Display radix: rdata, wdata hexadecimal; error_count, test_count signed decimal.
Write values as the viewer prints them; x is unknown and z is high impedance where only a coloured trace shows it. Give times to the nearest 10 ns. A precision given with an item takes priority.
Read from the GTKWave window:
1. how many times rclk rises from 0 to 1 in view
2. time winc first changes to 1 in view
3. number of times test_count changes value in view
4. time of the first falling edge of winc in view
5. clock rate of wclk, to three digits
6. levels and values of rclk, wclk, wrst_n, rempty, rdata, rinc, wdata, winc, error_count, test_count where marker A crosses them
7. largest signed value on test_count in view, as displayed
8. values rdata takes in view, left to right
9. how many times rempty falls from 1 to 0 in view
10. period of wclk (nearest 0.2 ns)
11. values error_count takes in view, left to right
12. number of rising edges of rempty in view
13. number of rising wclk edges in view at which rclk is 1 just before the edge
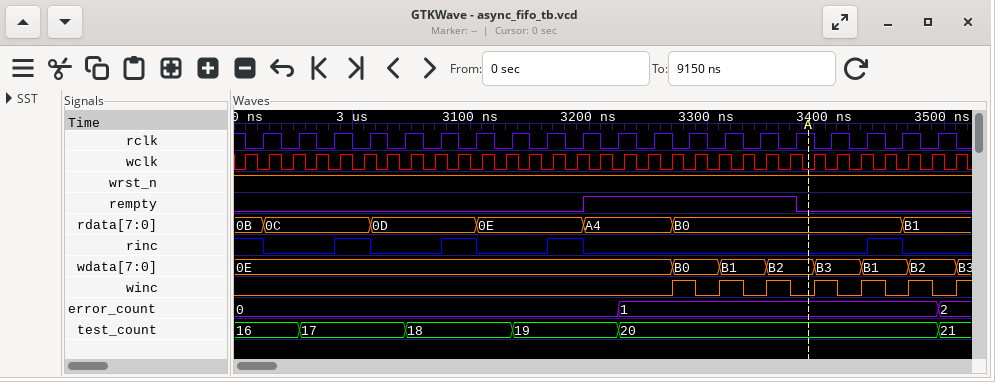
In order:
20
3270 ns
5
3290 ns
50.0 MHz
rclk=1, wclk=0, wrst_n=1, rempty=0, rdata=B0, rinc=0, wdata=B2, winc=0, error_count=1, test_count=20
21
0B, 0C, 0D, 0E, A4, B0, B1
1
20 ns
0, 1, 2
1
21
